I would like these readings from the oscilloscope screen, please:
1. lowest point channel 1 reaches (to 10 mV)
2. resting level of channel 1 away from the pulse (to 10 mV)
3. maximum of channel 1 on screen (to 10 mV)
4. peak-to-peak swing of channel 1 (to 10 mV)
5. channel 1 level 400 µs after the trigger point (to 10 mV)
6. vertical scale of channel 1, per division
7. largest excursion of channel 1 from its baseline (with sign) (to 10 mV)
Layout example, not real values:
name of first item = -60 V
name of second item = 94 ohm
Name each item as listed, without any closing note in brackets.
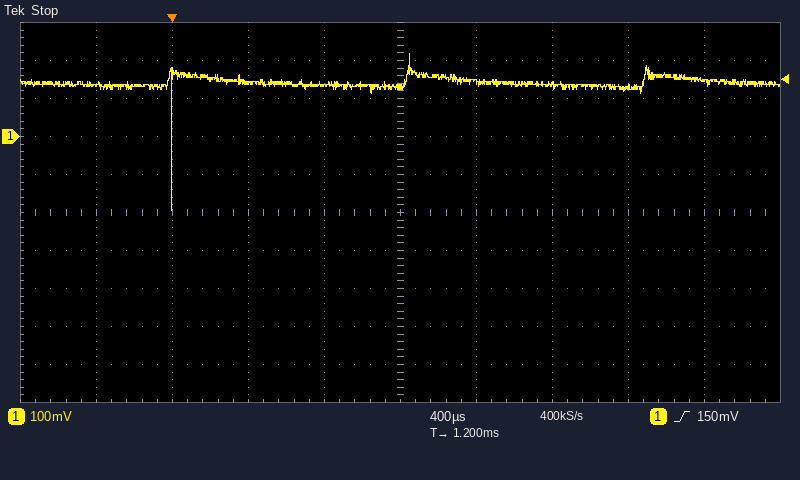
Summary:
lowest point channel 1 reaches = -190 mV
resting level of channel 1 away from the pulse = 140 mV
maximum of channel 1 on screen = 220 mV
peak-to-peak swing of channel 1 = 410 mV
channel 1 level 400 µs after the trigger point = 140 mV
vertical scale of channel 1, per division = 100 mV
largest excursion of channel 1 from its baseline (with sign) = -330 mV
